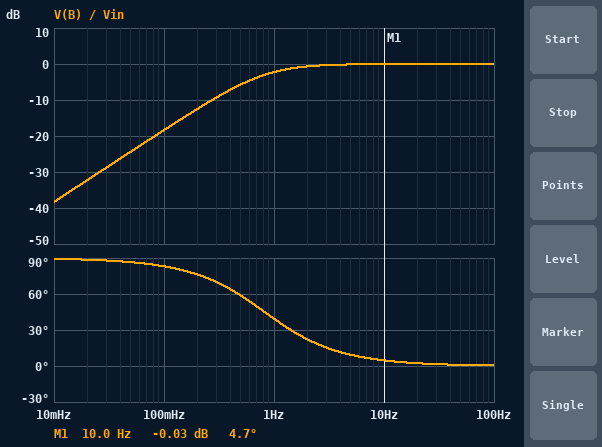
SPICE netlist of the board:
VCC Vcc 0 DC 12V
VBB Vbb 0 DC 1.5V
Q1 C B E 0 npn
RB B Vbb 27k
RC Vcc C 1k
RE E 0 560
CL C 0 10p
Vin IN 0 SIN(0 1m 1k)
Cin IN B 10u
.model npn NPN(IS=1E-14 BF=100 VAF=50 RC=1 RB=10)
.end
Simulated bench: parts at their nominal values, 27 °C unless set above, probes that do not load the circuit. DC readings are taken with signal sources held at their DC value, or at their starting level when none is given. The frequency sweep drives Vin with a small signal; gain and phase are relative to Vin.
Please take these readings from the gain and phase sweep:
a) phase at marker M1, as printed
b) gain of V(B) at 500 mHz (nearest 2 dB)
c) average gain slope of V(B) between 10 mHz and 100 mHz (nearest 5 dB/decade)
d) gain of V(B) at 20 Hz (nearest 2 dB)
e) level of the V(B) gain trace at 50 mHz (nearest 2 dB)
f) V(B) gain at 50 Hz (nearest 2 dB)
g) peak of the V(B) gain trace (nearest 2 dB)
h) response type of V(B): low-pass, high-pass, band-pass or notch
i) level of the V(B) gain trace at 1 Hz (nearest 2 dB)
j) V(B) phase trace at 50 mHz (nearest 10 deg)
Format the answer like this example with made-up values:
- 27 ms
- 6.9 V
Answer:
- 4.7 deg
- -6 dB
- 20 dB/decade
- 0 dB
- -24 dB
- 0 dB
- 0 dB
- high-pass
- -2 dB
- 90 deg
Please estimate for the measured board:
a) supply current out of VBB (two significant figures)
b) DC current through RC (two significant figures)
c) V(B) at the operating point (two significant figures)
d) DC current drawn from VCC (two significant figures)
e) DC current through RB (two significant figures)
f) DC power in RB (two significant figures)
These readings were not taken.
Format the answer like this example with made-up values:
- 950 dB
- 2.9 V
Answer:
- 9.0 µA
- 1.1 mA
- 1.3 V
- 1.1 mA
- 9.0 µA
- 2.2 µW
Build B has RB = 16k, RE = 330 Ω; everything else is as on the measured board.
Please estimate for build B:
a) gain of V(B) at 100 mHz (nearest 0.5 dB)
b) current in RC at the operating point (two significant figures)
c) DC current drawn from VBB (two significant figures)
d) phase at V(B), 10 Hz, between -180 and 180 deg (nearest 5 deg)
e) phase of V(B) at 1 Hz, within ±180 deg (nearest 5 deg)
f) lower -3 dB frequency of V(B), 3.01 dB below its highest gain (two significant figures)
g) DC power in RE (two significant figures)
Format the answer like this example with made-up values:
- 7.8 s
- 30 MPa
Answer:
- -23.0 dB
- 1.8 mA
- 15 µA
- 10 deg
- 55 deg
- 1.4 Hz
- 1.1 mW
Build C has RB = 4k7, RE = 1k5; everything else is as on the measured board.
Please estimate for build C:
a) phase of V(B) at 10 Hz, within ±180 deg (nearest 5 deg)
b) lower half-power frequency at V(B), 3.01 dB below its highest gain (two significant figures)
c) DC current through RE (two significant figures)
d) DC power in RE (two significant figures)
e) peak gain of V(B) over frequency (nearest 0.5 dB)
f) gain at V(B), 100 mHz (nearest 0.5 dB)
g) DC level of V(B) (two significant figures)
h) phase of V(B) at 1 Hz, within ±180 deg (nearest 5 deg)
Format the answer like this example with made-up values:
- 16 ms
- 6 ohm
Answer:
- 20 deg
- 3.5 Hz
- 560 µA
- 470 µW
- 0 dB
- -31.0 dB
- 1.5 V
- 75 deg
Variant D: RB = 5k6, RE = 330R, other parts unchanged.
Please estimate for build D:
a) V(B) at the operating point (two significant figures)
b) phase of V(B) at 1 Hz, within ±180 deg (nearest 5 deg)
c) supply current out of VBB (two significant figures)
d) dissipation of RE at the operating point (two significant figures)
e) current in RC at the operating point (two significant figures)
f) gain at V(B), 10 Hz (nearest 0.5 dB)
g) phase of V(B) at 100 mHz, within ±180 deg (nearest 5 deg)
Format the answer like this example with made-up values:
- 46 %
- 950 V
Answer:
- 1.4 V
- 75 deg
- 19 µA
- 1.6 mW
- 2.2 mA
- -0.5 dB
- 90 deg
